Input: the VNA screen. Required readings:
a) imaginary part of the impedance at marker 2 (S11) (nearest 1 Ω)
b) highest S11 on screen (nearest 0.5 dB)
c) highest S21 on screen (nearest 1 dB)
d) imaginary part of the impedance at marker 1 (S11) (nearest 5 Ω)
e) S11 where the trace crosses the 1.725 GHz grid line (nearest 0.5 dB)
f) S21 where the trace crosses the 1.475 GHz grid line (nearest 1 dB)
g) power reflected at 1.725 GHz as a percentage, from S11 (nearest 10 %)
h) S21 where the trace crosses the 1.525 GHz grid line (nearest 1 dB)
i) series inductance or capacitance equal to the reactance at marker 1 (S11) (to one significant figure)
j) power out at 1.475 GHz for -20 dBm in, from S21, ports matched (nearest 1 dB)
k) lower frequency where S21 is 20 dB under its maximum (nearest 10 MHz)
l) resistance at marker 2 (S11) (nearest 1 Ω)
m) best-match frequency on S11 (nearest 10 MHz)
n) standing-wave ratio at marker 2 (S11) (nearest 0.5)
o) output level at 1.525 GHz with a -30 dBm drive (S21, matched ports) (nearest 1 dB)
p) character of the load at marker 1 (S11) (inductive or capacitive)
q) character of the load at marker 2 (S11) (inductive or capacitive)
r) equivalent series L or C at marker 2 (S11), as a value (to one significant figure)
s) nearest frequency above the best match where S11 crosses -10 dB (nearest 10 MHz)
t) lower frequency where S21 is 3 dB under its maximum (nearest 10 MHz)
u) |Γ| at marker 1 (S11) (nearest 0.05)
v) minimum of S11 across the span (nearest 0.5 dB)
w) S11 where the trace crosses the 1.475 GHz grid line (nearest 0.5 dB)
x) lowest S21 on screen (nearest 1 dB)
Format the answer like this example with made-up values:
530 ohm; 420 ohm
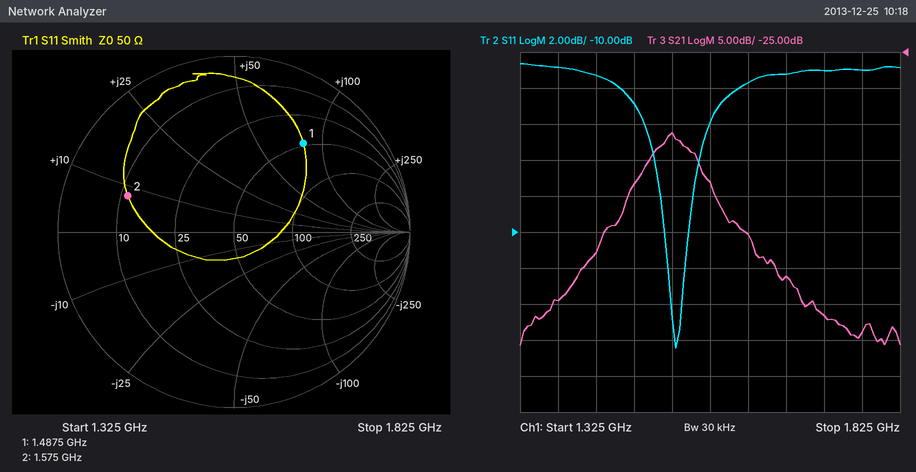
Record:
+8 Ω; -0.5 dB; -36 dB; +80 Ω; -1.0 dB; -43 dB; 80 %; -36 dB; 9 nH; -63 dBm; 1.40 GHz; 11 Ω; 1.53 GHz; 4.5; -66 dBm; inductive; inductive; 800 pH; 1.55 GHz; 1.50 GHz; 0.65; -16.5 dB; -3.0 dB; -66 dB
